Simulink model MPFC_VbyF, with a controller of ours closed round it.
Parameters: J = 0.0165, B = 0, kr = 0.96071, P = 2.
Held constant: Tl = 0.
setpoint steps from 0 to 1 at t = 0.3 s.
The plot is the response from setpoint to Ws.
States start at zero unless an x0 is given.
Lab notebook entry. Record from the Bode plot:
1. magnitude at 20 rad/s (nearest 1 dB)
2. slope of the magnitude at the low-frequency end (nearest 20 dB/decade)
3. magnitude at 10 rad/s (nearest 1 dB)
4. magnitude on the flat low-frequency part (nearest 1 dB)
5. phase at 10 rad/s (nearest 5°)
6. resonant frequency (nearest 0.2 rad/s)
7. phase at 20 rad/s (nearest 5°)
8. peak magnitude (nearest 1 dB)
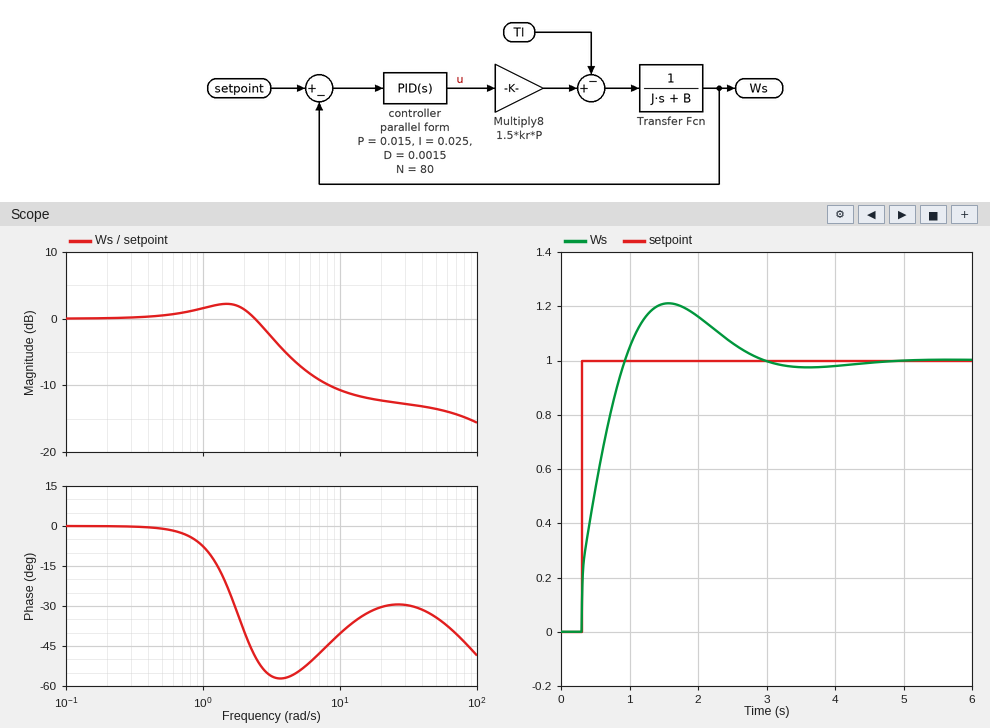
-12 dB
0 dB/decade
-11 dB
0 dB
-40°
1.4 rad/s
-30°
2 dB
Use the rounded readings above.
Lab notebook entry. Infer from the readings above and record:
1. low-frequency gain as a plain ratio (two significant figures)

1.0
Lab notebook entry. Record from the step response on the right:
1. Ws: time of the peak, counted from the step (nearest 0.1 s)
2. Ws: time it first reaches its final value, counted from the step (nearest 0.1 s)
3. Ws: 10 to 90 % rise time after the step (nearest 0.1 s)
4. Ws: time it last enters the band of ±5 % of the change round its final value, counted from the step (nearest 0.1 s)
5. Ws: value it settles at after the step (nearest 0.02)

1.3 s
0.6 s
0.5 s
2.3 s
1.00
